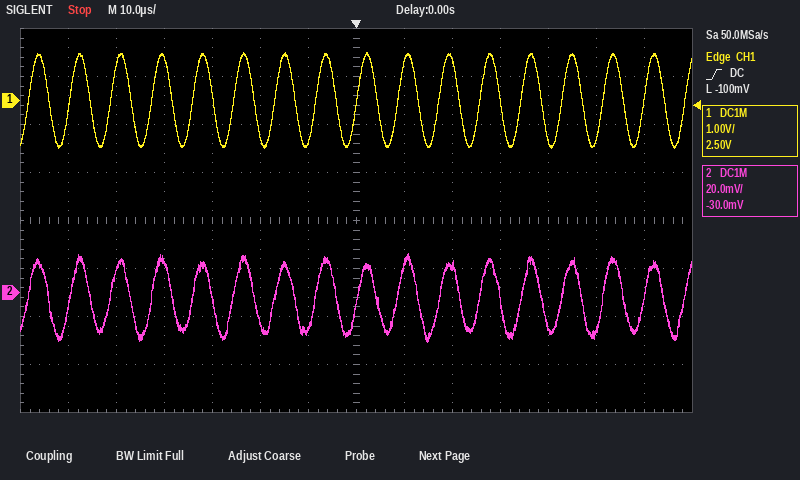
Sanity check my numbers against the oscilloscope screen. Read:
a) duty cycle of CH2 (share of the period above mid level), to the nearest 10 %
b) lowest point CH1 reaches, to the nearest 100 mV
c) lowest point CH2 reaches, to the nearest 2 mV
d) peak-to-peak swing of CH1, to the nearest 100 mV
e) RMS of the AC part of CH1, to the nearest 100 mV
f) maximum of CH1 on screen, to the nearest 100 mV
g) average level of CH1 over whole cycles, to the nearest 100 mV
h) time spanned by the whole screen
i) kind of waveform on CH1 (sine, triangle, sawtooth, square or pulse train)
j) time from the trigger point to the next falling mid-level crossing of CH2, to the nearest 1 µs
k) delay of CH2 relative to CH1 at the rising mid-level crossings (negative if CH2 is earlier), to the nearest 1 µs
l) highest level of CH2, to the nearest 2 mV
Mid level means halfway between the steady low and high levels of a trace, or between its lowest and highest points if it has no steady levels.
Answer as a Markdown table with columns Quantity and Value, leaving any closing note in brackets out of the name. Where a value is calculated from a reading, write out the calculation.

| Quantity | Value |
|---|---|
| duty cycle of CH2 (share of the period above mid level), to the nearest 10 % | 50 % |
| lowest point CH1 reaches, to the nearest 100 mV | -1.0 V |
| lowest point CH2 reaches, to the nearest 2 mV | -20 mV |
| peak-to-peak swing of CH1, to the nearest 100 mV | 1.0 V − (-1.0 V) = 2.0 V |
| RMS of the AC part of CH1, to the nearest 100 mV | 2.0 V / (2√2) ≈ 707 mV, so 700 mV to the nearest 100 mV |
| maximum of CH1 on screen, to the nearest 100 mV | 1.0 V |
| average level of CH1 over whole cycles, to the nearest 100 mV | (1.0 V + (-1.0 V)) / 2 ≈ 0.0 V |
| time spanned by the whole screen | 140 µs |
| kind of waveform on CH1 | sine |
| time from the trigger point to the next falling mid-level crossing of CH2, to the nearest 1 µs | 4 µs |
| delay of CH2 relative to CH1 at the rising mid-level crossings (negative if CH2 is earlier), to the nearest 1 µs | 0 µs |
| highest level of CH2, to the nearest 2 mV | 16 mV |
